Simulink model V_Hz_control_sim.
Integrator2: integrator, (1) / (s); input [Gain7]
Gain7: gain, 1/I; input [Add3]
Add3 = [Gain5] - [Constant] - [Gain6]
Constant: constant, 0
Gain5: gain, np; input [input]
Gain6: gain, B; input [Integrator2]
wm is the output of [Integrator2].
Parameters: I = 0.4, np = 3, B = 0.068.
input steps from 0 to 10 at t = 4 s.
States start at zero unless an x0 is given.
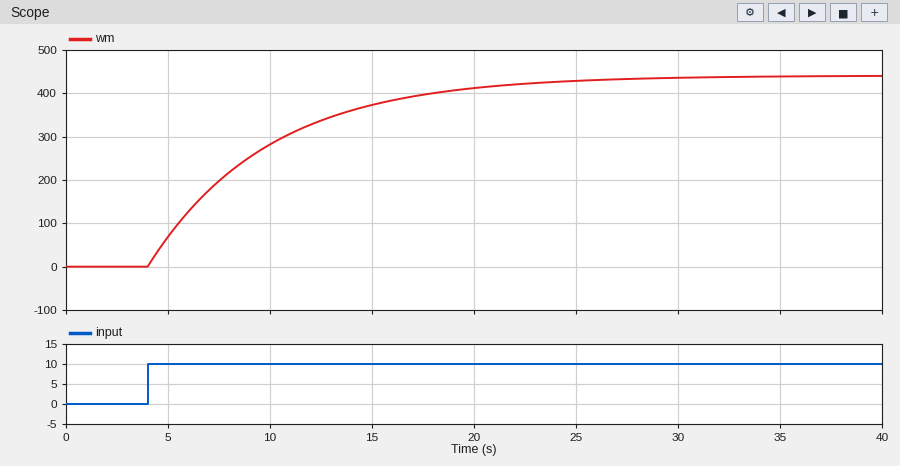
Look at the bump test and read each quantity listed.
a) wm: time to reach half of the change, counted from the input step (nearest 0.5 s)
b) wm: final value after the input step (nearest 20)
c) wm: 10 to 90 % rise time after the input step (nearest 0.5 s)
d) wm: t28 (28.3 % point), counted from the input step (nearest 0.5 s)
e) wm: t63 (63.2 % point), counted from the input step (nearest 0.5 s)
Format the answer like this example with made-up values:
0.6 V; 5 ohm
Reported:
4.0 s; 440; 13.0 s; 2.0 s; 6.0 s
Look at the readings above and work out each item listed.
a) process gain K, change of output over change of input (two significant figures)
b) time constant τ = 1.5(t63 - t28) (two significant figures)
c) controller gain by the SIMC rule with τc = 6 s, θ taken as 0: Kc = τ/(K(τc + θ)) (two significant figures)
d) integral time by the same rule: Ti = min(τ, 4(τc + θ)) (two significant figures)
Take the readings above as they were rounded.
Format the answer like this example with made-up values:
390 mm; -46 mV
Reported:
44; 6.0 s; 0.023; 6.0 s
